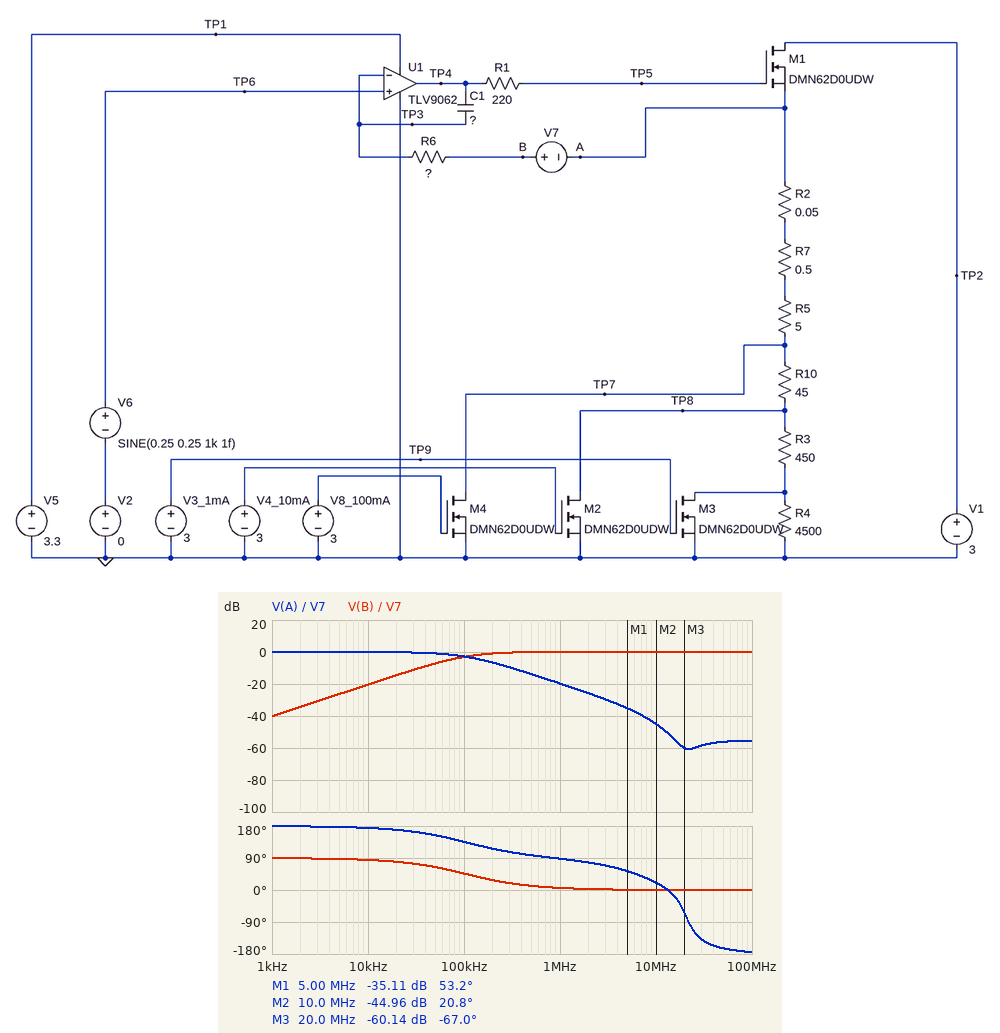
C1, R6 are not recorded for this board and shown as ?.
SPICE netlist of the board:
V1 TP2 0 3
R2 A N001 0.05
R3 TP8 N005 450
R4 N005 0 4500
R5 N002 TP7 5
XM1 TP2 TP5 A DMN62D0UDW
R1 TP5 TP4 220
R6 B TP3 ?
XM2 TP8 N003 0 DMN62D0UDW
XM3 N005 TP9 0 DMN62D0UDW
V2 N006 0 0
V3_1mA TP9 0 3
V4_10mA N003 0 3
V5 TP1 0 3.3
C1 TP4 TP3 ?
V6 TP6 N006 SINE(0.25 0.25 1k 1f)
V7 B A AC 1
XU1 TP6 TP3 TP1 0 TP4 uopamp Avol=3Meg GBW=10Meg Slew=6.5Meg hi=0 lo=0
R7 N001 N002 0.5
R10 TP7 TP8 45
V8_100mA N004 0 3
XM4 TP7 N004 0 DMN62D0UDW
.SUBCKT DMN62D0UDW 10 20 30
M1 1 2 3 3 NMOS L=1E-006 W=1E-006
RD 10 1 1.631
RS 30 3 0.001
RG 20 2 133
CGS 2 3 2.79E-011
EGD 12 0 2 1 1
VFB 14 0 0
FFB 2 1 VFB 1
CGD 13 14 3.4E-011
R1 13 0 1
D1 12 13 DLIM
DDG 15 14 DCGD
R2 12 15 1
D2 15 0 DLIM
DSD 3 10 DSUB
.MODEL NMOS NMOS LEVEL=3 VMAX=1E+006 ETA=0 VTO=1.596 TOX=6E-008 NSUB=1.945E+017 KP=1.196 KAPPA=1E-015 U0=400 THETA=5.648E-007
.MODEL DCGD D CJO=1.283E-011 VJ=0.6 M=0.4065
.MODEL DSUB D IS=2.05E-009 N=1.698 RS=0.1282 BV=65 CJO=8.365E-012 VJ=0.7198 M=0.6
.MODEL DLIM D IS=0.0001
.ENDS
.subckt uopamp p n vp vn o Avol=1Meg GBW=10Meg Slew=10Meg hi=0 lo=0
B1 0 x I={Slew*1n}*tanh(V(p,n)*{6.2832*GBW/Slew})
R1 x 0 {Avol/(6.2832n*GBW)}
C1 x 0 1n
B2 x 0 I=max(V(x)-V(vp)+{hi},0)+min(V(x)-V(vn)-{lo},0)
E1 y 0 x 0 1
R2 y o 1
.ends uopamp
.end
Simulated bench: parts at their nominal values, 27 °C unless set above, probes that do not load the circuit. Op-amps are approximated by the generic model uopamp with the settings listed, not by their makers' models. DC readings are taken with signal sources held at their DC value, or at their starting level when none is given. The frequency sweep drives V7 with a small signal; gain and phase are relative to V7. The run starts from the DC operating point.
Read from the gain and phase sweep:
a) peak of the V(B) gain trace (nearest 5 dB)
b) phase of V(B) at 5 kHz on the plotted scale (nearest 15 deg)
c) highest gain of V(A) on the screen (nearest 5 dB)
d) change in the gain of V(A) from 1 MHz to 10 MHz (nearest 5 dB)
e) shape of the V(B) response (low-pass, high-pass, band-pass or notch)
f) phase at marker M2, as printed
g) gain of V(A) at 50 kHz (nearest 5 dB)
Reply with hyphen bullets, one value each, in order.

- 0 dB
- 90 deg
- 0 dB
- -25 dB
- high-pass
- 20.8 deg
- 0 dB
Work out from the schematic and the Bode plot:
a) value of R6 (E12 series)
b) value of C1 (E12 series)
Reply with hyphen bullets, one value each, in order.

- 3.3 kΩ
- 270 pF
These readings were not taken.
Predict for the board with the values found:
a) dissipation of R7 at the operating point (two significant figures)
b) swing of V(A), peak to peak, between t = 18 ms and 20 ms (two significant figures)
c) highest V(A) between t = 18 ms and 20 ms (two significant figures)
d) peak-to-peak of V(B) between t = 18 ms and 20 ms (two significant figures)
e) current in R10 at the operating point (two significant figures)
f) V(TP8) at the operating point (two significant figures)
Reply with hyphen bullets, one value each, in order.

- 530 µW
- 500 mV
- 500 mV
- 500 mV
- 1.5 mA
- 3.3 mV
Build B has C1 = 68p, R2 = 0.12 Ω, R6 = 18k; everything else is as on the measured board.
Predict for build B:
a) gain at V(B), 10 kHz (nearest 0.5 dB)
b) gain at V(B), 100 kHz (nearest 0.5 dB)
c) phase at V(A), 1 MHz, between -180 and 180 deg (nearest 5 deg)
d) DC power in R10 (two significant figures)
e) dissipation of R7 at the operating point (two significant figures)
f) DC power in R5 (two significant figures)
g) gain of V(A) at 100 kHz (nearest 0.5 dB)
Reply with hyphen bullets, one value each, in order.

- -17.5 dB
- -2.0 dB
- 85 deg
- 96 µW
- 520 µW
- 5.2 mW
- -4.5 dB
